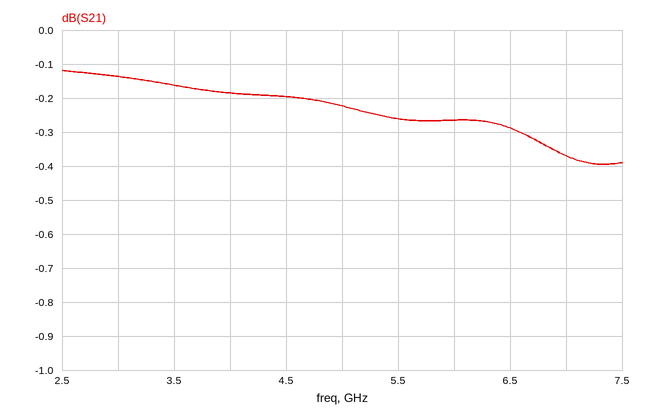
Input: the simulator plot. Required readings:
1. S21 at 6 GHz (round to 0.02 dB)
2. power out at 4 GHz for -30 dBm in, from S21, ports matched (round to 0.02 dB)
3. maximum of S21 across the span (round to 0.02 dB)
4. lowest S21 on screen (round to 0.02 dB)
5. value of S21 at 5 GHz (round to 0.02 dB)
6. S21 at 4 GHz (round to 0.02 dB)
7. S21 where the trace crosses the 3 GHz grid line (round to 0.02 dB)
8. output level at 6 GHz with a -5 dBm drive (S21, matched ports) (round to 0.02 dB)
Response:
-0.26 dB
-30.18 dBm
-0.12 dB
-0.40 dB
-0.22 dB
-0.18 dB
-0.14 dB
-5.26 dBm
